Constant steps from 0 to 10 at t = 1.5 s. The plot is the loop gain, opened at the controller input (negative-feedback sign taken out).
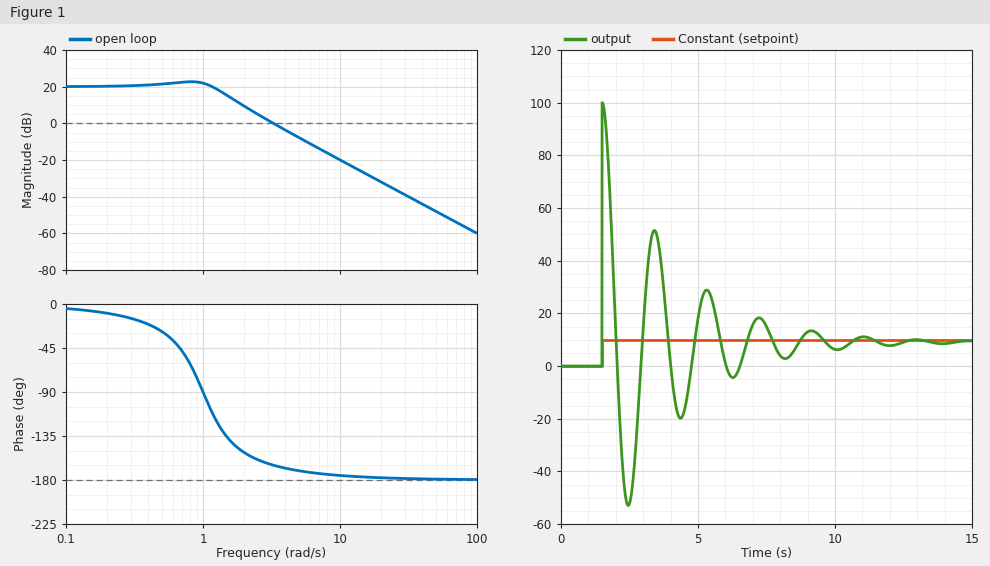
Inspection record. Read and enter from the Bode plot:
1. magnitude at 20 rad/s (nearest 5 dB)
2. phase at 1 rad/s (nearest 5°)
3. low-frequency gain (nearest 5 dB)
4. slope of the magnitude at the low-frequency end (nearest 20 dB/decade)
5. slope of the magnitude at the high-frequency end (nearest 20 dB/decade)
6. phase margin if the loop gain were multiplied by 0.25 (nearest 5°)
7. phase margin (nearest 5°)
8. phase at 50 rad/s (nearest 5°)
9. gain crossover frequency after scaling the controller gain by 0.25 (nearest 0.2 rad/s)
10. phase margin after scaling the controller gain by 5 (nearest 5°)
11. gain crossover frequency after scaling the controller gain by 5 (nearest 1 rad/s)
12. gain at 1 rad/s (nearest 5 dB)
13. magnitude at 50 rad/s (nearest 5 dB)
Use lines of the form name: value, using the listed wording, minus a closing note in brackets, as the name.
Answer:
magnitude at 20 rad/s: -30 dB
phase at 1 rad/s: -90°
low-frequency gain: 20 dB
slope of the magnitude at the low-frequency end: 0 dB/decade
slope of the magnitude at the high-frequency end: -40 dB/decade
phase margin if the loop gain were multiplied by 0.25: 35°
phase margin: 15°
phase at 50 rad/s: -180°
gain crossover frequency after scaling the controller gain by 0.25: 1.8 rad/s
phase margin after scaling the controller gain by 5: 5°
gain crossover frequency after scaling the controller gain by 5: 7 rad/s
gain at 1 rad/s: 20 dB
magnitude at 50 rad/s: -50 dB
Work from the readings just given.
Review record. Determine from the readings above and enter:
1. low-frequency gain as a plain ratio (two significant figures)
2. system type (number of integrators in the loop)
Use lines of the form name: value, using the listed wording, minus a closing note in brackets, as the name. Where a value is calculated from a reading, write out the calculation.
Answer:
low-frequency gain as a plain ratio: 10^(20 / 20) = 10
system type: 0
